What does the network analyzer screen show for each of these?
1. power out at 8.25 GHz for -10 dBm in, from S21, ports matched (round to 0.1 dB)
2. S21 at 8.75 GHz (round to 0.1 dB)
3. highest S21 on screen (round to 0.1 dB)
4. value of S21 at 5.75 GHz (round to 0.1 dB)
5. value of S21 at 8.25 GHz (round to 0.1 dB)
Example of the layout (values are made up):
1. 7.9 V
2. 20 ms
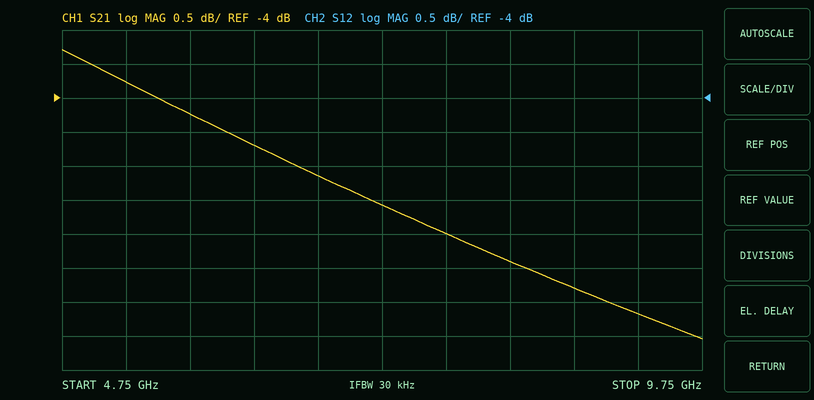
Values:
1. -16.4 dBm
2. -6.8 dB
3. -3.3 dB
4. -4.2 dB
5. -6.4 dB
